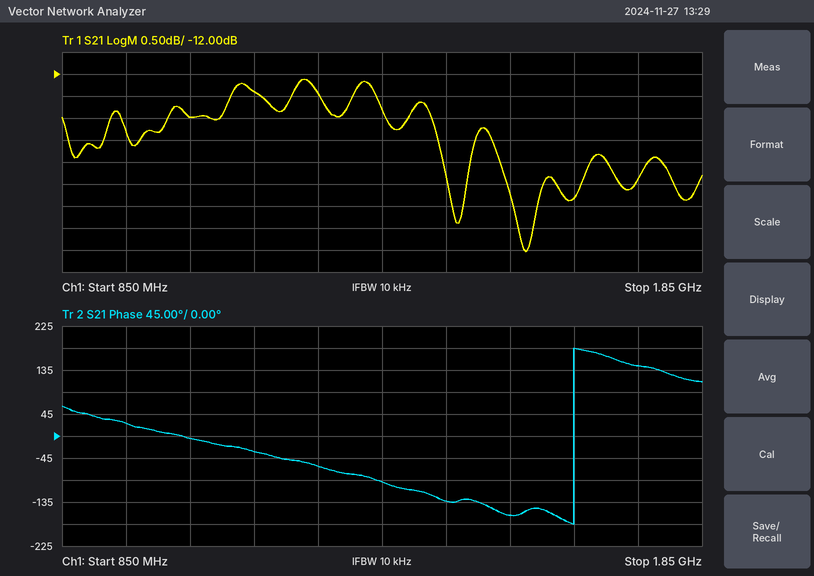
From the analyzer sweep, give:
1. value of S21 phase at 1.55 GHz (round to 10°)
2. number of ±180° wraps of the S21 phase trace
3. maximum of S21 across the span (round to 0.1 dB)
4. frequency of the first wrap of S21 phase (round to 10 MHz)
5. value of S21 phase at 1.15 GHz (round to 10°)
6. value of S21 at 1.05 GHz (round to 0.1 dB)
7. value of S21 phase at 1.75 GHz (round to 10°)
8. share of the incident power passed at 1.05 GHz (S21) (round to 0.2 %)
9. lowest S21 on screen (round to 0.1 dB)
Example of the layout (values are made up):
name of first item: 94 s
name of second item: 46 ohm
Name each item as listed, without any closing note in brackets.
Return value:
value of S21 phase at 1.55 GHz: -160°
number of ±180° wraps of the S21 phase trace: 1
maximum of S21 across the span: -12.1 dB
frequency of the first wrap of S21 phase: 1.65 GHz
value of S21 phase at 1.15 GHz: -30°
value of S21 at 1.05 GHz: -13.0 dB
value of S21 phase at 1.75 GHz: 140°
share of the incident power passed at 1.05 GHz (S21): 5.0 %
lowest S21 on screen: -16.0 dB
